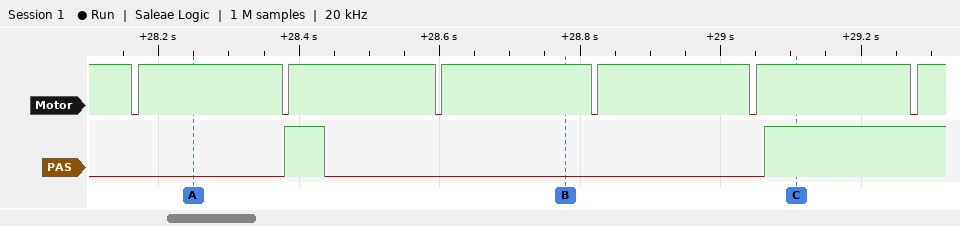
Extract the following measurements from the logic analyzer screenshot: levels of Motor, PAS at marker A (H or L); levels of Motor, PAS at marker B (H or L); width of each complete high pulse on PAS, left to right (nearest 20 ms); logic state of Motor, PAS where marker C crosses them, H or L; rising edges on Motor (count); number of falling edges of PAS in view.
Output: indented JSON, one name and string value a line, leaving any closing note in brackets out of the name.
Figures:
{
  "levels of Motor, PAS at marker A": "Motor=H, PAS=L",
  "levels of Motor, PAS at marker B": "Motor=H, PAS=L",
  "width of each complete high pulse on PAS, left to right": "60 ms",
  "logic state of Motor, PAS where marker C crosses them, H or L": "Motor=H, PAS=H",
  "rising edges on Motor": "6",
  "number of falling edges of PAS in view": "1"
}
